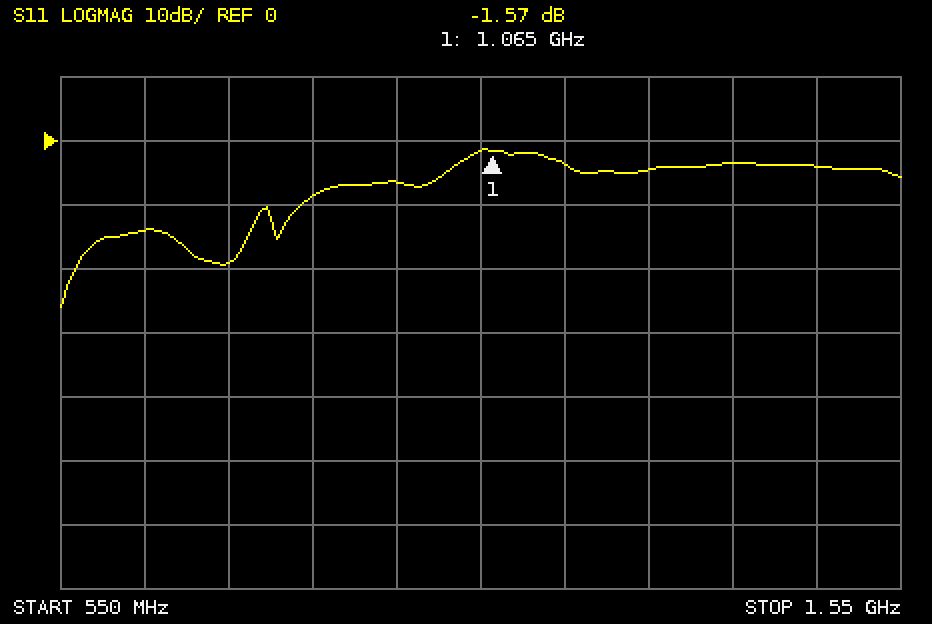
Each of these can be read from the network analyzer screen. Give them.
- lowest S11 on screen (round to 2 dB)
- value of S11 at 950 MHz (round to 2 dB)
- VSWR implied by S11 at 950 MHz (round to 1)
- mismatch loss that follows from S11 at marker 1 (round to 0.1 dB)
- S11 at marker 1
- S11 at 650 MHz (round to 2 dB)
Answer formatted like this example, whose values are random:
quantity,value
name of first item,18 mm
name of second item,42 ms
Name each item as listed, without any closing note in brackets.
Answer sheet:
quantity,value
lowest S11 on screen,-26 dB
value of S11 at 950 MHz,-6 dB
VSWR implied by S11 at 950 MHz,3
mismatch loss that follows from S11 at marker 1,5.2 dB
S11 at marker 1,-1.57 dB
S11 at 650 MHz,-14 dB
